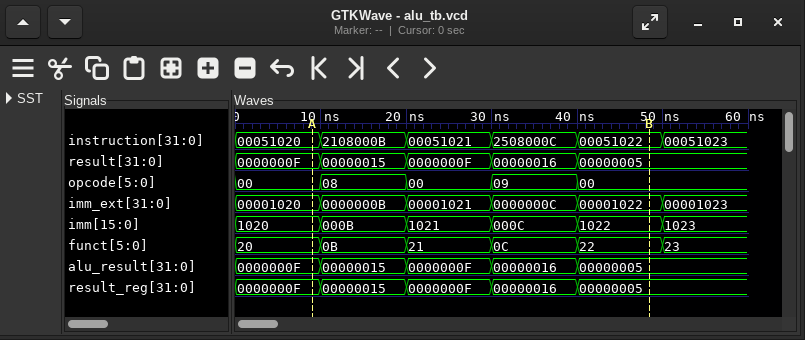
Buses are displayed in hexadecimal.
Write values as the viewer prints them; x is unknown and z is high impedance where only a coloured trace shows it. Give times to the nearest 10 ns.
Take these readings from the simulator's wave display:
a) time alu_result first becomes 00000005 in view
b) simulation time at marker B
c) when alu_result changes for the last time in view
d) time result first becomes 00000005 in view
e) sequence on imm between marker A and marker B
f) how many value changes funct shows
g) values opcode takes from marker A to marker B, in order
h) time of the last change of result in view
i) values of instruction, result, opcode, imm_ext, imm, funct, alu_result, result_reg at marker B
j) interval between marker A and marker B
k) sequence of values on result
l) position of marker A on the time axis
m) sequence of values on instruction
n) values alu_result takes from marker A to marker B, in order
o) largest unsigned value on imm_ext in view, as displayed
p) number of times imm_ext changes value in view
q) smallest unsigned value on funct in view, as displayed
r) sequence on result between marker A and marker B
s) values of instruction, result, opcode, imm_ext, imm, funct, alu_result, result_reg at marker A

40 ns
50 ns
40 ns
40 ns
1020, 000B, 1021, 000C, 1022
5
00, 08, 00, 09, 00
40 ns
instruction=00051022, result=00000005, opcode=00, imm_ext=00001022, imm=1022, funct=22, alu_result=00000005, result_reg=00000005
40 ns
0000000F, 00000015, 0000000F, 00000016, 00000005
10 ns
00051020, 2108000B, 00051021, 2508000C, 00051022, 00051023
0000000F, 00000015, 0000000F, 00000016, 00000005
00001023
5
0B
0000000F, 00000015, 0000000F, 00000016, 00000005
instruction=00051020, result=0000000F, opcode=00, imm_ext=00001020, imm=1020, funct=20, alu_result=0000000F, result_reg=0000000F
